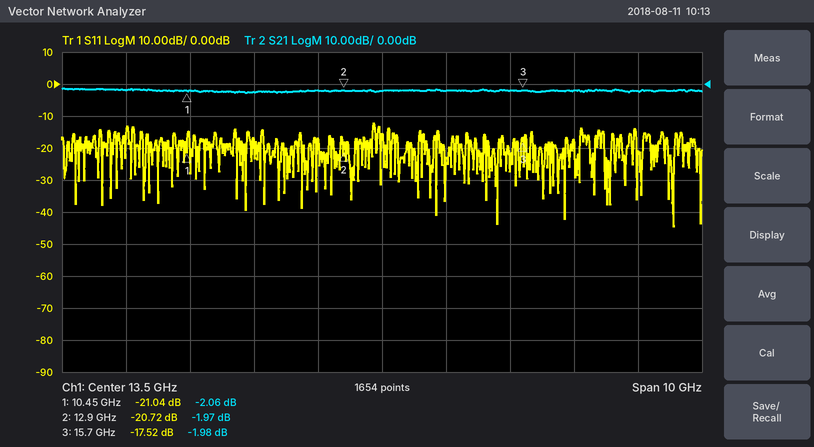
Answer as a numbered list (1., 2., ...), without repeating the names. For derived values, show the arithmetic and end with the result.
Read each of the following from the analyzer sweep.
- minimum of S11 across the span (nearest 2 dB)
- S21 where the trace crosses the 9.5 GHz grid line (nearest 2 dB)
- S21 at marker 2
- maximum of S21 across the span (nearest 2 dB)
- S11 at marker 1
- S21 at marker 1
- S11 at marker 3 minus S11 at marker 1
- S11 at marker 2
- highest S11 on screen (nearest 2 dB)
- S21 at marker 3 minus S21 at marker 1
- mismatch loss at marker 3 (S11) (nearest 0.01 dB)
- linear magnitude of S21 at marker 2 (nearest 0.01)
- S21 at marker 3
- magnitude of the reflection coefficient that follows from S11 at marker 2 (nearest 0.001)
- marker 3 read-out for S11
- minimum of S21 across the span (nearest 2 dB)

1. -44 dB
2. -2 dB
3. -1.97 dB
4. -2 dB
5. -21.04 dB
6. -2.06 dB
7. -17.52 − (-21.04) = 3.52 dB
8. -20.72 dB
9. -12 dB
10. -1.98 − (-2.06) = 0.08 dB
11. −10 log10(1 − 10^(-17.52/10)) ≈ 0.08 dB
12. 10^(-1.97/20) ≈ 0.80
13. -1.98 dB
14. 10^(-20.72/20) ≈ 0.092
15. -17.52 dB
16. -2 dB
